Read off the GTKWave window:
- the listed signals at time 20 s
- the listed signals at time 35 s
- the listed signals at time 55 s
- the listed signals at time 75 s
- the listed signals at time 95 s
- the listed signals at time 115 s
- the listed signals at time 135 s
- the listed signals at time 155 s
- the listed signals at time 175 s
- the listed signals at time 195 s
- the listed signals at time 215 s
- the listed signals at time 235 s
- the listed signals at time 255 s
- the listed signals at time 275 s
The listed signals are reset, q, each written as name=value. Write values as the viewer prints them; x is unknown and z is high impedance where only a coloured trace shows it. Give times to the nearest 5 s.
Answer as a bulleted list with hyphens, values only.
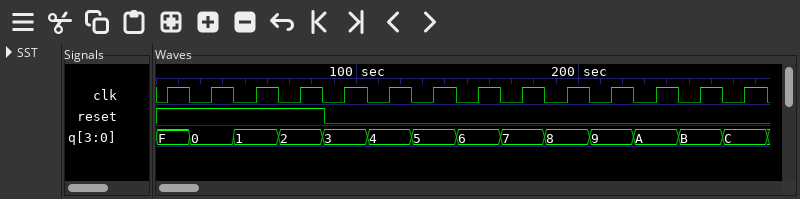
- reset=1, q=F
- reset=1, q=0
- reset=1, q=1
- reset=1, q=2
- reset=0, q=3
- reset=0, q=4
- reset=0, q=5
- reset=0, q=6
- reset=0, q=7
- reset=0, q=8
- reset=0, q=9
- reset=0, q=A
- reset=0, q=B
- reset=0, q=C
